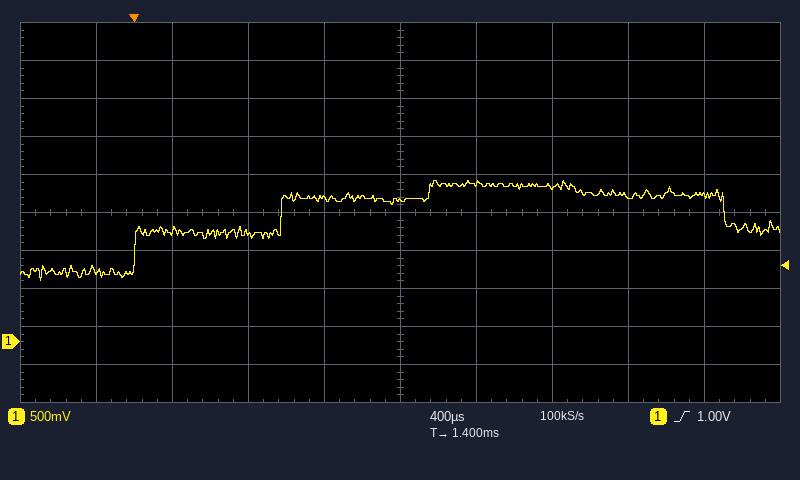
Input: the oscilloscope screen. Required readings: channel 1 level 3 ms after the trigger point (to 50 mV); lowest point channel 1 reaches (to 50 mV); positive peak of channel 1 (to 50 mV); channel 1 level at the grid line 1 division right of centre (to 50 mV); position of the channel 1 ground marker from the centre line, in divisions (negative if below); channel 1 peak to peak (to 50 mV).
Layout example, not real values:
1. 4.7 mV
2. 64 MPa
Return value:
1. 1.90 V
2. 800 mV
3. 2.10 V
4. 2.10 V
5. -3.4 div
6. 1.30 V
